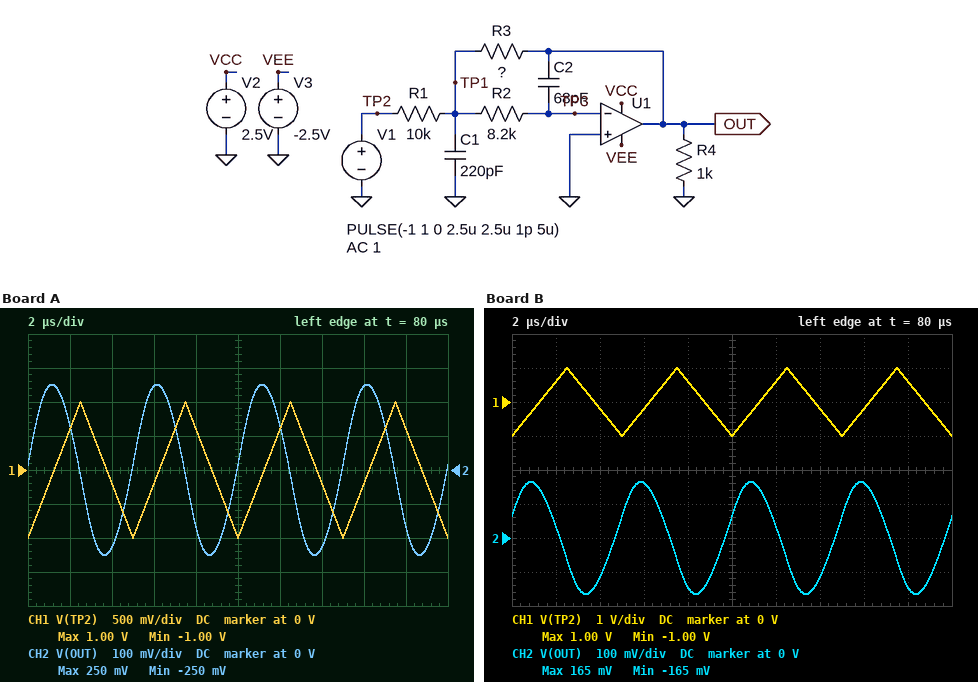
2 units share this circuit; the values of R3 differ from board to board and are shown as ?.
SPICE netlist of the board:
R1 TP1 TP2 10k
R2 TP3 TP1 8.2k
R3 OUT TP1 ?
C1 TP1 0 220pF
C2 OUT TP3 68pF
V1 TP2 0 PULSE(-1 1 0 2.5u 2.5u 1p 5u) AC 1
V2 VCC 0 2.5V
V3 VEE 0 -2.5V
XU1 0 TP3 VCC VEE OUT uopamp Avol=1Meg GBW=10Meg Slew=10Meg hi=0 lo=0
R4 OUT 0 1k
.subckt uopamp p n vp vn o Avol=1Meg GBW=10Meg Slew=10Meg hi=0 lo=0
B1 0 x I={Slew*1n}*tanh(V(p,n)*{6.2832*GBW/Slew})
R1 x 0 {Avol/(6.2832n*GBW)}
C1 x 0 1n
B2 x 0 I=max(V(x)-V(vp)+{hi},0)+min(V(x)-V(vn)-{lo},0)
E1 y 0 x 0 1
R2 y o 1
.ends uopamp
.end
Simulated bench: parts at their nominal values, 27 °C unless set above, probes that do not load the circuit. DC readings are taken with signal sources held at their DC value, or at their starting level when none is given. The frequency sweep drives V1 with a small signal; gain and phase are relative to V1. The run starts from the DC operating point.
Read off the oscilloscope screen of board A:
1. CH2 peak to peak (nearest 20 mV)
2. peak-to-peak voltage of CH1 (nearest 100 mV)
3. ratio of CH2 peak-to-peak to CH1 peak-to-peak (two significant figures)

500 mV
2.0 V
0.25
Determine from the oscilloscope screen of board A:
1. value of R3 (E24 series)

4.3 kΩ
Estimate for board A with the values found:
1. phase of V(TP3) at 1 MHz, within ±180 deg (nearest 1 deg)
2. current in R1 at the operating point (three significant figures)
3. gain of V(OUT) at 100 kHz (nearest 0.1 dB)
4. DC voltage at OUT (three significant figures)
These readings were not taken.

-77 deg
100 µA
-7.7 dB
430 mV
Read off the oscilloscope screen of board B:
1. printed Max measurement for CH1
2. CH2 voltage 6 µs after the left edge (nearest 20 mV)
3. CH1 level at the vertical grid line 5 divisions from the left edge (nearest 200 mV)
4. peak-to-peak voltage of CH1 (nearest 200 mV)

1.00 V
160 mV
-1.0 V
2.0 V
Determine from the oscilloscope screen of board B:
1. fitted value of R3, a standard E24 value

2.4 kΩ
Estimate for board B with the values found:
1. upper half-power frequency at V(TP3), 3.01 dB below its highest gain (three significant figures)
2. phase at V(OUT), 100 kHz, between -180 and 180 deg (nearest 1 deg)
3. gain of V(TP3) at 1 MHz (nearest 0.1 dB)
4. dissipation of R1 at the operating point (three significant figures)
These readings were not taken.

591 kHz
148 deg
-54.2 dB
100 µW
